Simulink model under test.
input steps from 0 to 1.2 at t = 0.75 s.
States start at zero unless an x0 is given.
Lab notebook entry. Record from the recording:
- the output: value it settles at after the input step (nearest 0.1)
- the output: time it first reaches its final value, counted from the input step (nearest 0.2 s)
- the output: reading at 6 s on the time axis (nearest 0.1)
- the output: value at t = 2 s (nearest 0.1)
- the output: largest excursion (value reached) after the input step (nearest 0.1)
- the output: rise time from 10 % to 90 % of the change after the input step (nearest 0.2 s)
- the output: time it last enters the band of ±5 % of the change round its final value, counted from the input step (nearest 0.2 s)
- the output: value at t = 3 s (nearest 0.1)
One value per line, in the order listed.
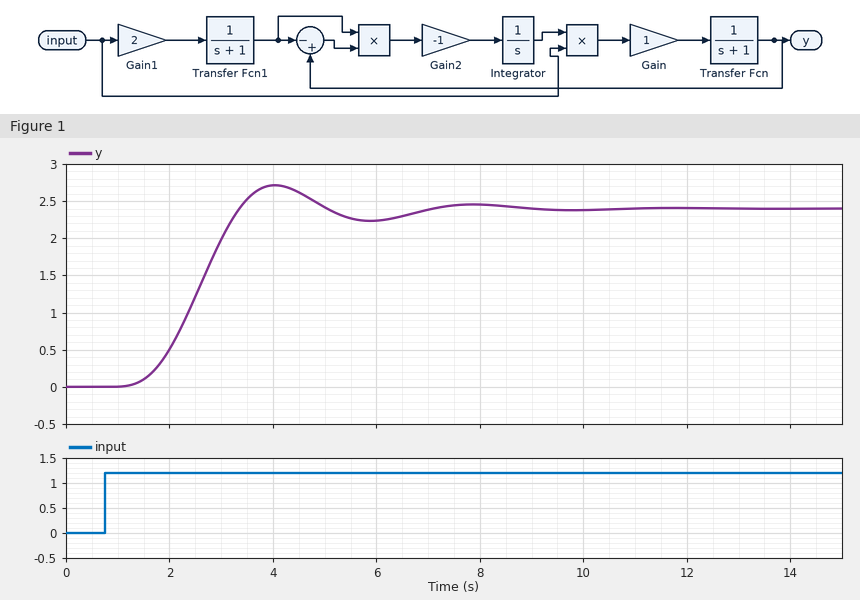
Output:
2.4
2.6 s
2.2
0.5
2.7
1.4 s
5.6 s
2.0
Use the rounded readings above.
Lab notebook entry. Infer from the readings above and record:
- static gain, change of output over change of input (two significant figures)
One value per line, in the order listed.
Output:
2.0
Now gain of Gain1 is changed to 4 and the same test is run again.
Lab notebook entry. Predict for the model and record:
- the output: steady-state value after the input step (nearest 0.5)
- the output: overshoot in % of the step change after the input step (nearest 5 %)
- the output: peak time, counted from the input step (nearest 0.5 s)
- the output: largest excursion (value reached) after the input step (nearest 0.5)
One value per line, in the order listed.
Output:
5.0
10 %
2.5 s
5.5
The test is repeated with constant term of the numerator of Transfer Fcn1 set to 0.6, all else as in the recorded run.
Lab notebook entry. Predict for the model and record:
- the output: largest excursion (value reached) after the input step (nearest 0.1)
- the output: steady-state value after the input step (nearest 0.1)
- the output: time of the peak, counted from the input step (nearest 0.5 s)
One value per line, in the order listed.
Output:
1.6
1.4
4.0 s
